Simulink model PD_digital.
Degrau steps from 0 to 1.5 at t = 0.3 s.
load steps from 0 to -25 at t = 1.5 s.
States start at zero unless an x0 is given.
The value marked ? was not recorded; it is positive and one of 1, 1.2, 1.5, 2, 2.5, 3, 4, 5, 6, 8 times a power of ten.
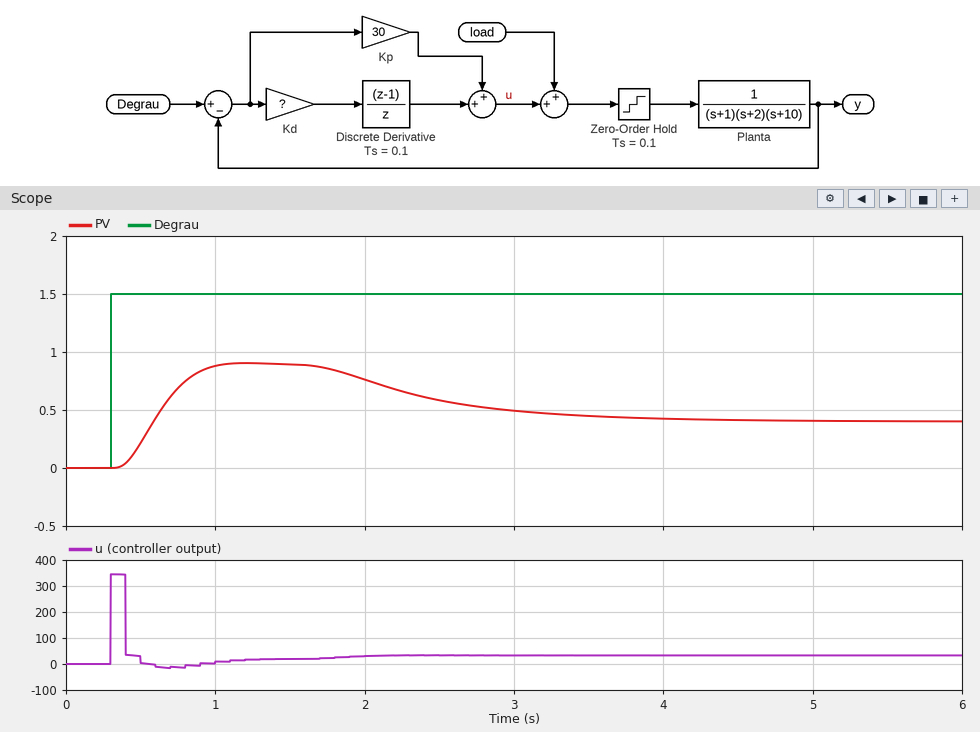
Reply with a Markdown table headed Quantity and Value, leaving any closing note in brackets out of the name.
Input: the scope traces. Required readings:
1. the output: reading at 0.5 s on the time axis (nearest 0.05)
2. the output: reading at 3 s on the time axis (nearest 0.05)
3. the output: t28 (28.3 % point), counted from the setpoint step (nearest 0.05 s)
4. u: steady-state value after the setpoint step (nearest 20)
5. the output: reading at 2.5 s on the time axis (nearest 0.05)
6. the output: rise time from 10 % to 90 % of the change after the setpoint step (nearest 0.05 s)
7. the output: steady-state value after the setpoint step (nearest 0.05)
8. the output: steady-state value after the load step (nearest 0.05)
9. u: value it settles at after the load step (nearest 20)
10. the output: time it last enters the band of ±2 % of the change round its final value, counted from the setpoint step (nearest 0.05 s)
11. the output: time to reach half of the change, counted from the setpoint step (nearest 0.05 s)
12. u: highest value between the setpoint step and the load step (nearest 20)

| Quantity | Value |
|---|---|
| the output: reading at 0.5 s on the time axis | 0.20 |
| the output: reading at 3 s on the time axis | 0.50 |
| the output: t28 (28.3 % point), counted from the setpoint step | 0.20 s |
| u: steady-state value after the setpoint step | 20 |
| the output: reading at 2.5 s on the time axis | 0.60 |
| the output: rise time from 10 % to 90 % of the change after the setpoint step | 0.45 s |
| the output: steady-state value after the setpoint step | 0.90 |
| the output: steady-state value after the load step | 0.40 |
| u: value it settles at after the load step | 40 |
| the output: time it last enters the band of ±2 % of the change round its final value, counted from the setpoint step | 0.70 s |
| the output: time to reach half of the change, counted from the setpoint step | 0.30 s |
| u: highest value between the setpoint step and the load step | 340 |
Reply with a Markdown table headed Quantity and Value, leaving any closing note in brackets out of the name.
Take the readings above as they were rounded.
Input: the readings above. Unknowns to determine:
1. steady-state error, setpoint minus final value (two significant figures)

| Quantity | Value |
|---|---|
| steady-state error, setpoint minus final value | 0.60 |
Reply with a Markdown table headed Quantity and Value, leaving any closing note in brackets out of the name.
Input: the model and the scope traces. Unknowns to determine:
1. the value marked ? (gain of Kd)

| Quantity | Value |
|---|---|
| the value marked ? | 200 |
